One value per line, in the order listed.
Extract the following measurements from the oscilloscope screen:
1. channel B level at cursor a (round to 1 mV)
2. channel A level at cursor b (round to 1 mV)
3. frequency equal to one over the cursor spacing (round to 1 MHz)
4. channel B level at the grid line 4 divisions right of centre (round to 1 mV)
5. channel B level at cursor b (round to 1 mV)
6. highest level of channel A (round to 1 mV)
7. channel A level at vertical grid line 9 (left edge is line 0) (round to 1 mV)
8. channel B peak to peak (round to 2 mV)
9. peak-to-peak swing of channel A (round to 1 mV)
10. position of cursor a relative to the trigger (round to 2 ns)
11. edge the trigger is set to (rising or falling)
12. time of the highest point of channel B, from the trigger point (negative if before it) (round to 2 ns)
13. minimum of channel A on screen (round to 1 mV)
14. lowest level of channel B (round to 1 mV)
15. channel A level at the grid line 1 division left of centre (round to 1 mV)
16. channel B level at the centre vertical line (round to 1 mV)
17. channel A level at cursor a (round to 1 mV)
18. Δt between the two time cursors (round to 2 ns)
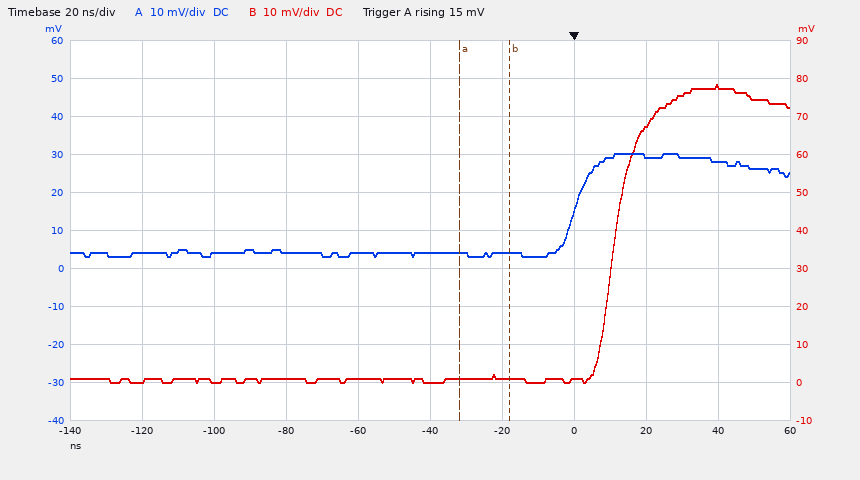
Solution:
1 mV
4 mV
71 MHz
78 mV
1 mV
30 mV
28 mV
78 mV
27 mV
-32 ns
rising
+40 ns
3 mV
0 mV
4 mV
0 mV
4 mV
14 ns
